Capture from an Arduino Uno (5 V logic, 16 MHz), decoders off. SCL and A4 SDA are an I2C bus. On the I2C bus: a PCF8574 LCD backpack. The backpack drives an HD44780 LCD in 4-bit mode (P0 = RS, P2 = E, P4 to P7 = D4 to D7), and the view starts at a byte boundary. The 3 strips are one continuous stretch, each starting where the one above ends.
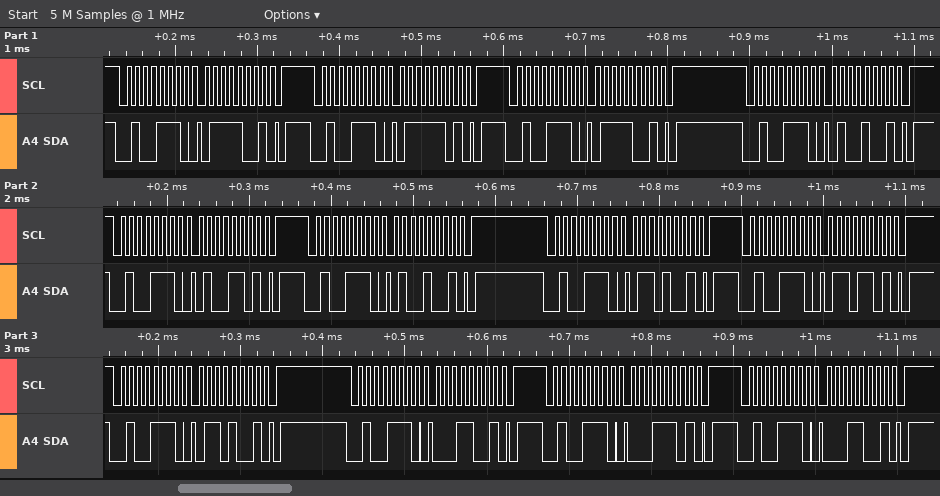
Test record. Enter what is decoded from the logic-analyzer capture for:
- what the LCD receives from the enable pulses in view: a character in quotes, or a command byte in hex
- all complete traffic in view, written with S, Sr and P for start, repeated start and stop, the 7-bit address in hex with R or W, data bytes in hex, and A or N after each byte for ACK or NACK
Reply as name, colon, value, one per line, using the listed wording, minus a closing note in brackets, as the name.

what the LCD receives from the enable pulses in view: a character in quotes, or a command byte in hex: 't' 'a'
all complete traffic in view, written with S, Sr and P for start, repeated start and stop, the 7-bit address in hex with R or W, data bytes in hex, and A or N after each byte for ACK or NACK: S 27W A 79 A P S 27W A 7D A P S 27W A 79 A P S 27W A 49 A P S 27W A 4D A P S 27W A 49 A P S 27W A 69 A P S 27W A 6D A P S 27W A 69 A P S 27W A 19 A P S 27W A 1D A P S 27W A 19 A P
